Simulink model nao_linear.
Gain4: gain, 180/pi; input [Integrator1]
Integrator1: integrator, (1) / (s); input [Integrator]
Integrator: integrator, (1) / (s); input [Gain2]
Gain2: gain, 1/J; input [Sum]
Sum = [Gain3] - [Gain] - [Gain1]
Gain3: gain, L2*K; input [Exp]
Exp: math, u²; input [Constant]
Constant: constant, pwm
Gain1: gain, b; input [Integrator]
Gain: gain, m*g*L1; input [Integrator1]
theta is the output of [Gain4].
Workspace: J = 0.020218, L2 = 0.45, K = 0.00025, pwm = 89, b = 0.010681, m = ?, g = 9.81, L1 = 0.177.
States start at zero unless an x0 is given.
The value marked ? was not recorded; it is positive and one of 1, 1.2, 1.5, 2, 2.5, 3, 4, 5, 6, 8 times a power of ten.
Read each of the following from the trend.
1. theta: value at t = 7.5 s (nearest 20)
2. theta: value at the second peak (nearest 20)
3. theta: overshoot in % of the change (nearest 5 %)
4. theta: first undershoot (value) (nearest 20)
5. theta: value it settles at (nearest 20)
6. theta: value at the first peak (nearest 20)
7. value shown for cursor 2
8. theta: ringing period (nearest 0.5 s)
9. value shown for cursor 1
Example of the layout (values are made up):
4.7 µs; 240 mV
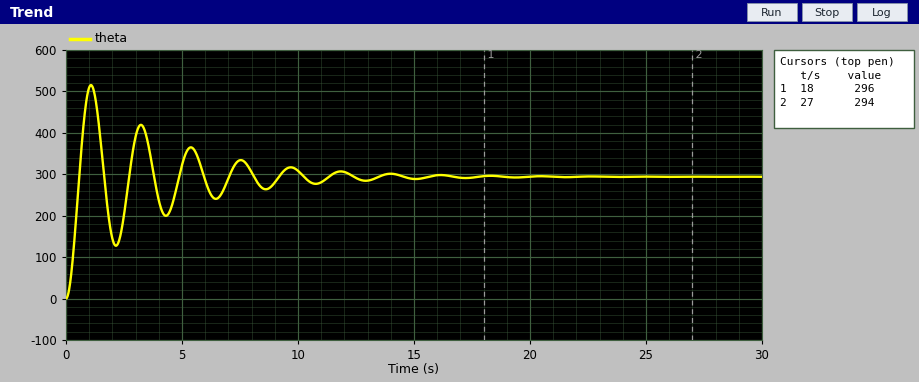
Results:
340; 420; 75 %; 120; 300; 520; 294; 2.0 s; 296
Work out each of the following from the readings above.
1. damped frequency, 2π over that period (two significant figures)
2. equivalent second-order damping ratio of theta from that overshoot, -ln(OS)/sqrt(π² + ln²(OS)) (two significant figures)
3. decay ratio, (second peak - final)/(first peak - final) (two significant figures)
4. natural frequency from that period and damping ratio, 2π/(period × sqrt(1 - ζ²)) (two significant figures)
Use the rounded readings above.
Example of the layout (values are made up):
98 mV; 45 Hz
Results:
3.1 rad/s; 0.091; 0.55; 3.2 rad/s
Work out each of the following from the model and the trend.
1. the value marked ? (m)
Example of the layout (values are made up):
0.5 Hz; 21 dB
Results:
0.1
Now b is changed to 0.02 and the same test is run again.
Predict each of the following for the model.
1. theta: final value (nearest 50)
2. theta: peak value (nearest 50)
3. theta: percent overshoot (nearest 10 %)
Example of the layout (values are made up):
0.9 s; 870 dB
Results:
300; 450; 60 %
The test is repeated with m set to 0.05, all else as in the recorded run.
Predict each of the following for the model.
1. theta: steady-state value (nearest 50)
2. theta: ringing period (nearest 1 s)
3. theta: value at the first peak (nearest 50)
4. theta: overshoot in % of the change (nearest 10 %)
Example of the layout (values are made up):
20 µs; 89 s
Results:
600; 3 s; 1000; 70 %
